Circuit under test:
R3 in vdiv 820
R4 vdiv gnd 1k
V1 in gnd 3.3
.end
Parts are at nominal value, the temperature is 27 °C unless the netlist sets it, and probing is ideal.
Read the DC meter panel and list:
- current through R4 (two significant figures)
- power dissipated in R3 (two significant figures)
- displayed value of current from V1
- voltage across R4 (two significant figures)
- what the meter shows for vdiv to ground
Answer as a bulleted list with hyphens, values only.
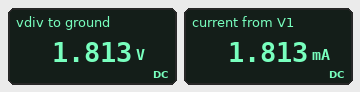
- 1.8 mA
- 2.7 mW
- 1.813 mA
- 1.8 V
- 1.813 V
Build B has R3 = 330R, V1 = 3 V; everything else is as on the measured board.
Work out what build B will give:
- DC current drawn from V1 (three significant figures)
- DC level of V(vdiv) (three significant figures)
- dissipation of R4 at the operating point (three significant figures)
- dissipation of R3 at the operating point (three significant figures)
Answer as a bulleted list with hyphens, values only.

- 2.26 mA
- 2.26 V
- 5.09 mW
- 1.68 mW
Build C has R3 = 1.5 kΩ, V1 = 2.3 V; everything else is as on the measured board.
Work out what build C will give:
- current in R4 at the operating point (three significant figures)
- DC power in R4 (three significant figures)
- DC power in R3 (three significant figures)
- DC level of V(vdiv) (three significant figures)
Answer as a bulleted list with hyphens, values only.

- 920 µA
- 846 µW
- 1.27 mW
- 920 mV
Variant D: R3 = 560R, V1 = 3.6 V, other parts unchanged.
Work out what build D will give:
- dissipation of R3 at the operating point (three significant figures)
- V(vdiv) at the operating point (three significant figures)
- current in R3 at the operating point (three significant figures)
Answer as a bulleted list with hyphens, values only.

- 2.98 mW
- 2.31 V
- 2.31 mA
